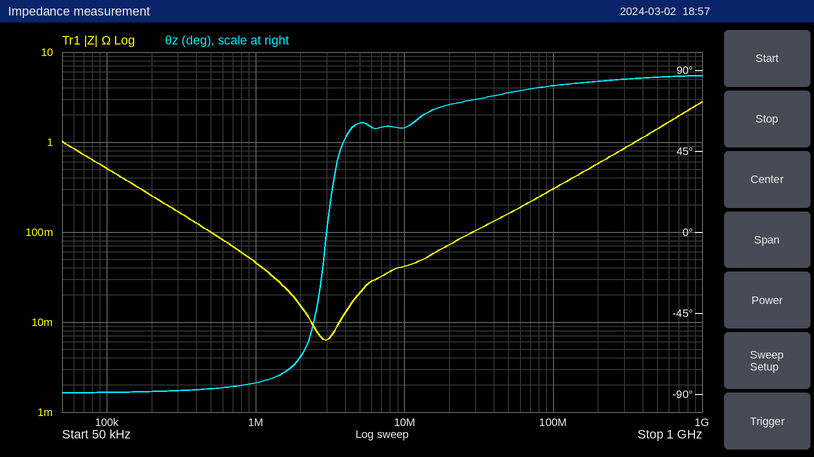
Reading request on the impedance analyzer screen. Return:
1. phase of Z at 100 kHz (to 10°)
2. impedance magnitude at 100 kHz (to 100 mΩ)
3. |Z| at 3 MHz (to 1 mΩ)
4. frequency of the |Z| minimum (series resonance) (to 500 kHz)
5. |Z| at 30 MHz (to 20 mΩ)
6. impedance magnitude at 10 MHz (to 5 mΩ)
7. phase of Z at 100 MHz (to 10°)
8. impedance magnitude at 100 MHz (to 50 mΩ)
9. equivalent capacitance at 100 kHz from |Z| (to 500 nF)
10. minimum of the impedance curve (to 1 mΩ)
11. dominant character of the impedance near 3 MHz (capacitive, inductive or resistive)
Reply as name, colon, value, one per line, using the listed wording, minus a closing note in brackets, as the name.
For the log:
phase of Z at 100 kHz: -90°
impedance magnitude at 100 kHz: 500 mΩ
|Z| at 3 MHz: 6 mΩ
frequency of the |Z| minimum (series resonance): 3.0 MHz
|Z| at 30 MHz: 100 mΩ
impedance magnitude at 10 MHz: 40 mΩ
phase of Z at 100 MHz: 80°
impedance magnitude at 100 MHz: 300 mΩ
equivalent capacitance at 100 kHz from |Z|: 3.0 µF
minimum of the impedance curve: 6 mΩ
dominant character of the impedance near 3 MHz: resistive
